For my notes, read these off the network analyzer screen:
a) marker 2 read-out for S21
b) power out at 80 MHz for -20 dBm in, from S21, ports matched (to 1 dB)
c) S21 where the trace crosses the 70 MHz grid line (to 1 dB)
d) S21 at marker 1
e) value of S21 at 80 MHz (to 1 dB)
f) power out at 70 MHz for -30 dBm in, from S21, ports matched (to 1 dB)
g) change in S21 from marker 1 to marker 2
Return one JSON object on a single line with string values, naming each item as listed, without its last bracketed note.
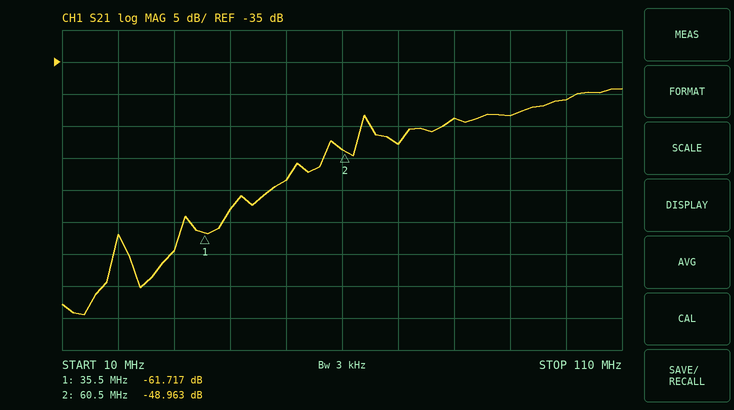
{"marker 2 read-out for S21": "-48.963 dB", "power out at 80 MHz for -20 dBm in, from S21, ports matched": "-64 dBm", "S21 where the trace crosses the 70 MHz grid line": "-48 dB", "S21 at marker 1": "-61.717 dB", "value of S21 at 80 MHz": "-44 dB", "power out at 70 MHz for -30 dBm in, from S21, ports matched": "-78 dBm", "change in S21 from marker 1 to marker 2": "12.754 dB"}
